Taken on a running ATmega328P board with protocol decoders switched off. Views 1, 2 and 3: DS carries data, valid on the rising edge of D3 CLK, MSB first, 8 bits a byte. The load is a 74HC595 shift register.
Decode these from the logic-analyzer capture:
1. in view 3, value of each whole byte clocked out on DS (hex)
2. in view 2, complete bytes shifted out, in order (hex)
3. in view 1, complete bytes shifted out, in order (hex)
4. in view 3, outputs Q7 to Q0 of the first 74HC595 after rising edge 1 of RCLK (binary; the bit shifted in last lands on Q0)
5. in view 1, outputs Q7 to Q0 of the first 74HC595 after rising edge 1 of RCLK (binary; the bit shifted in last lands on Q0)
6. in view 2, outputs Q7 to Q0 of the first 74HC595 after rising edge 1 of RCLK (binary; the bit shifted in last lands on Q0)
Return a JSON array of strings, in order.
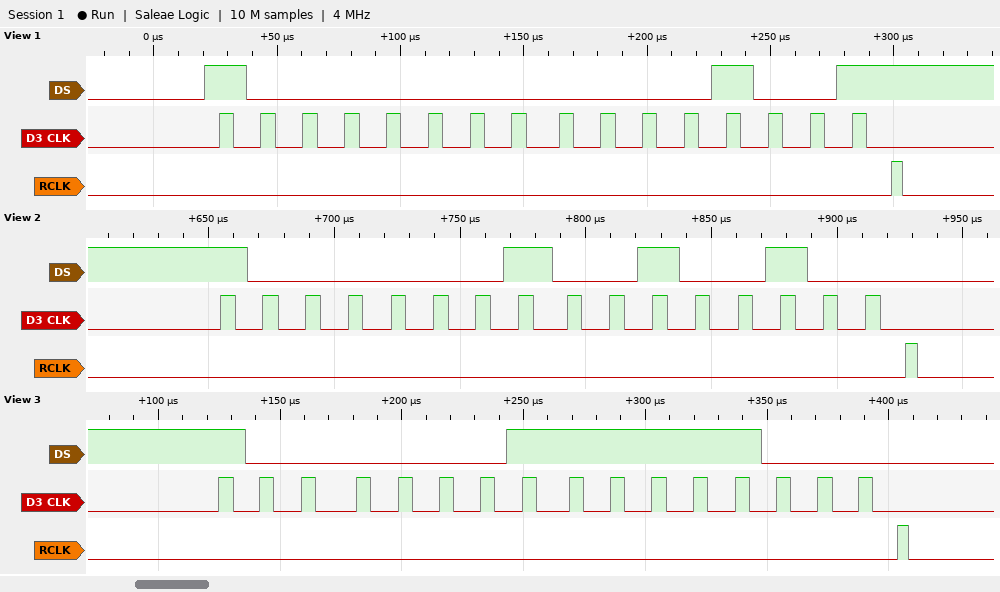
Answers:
["81 F8", "0x81 0x24", "80 09", "11111000", "00001001", "00100100"]
